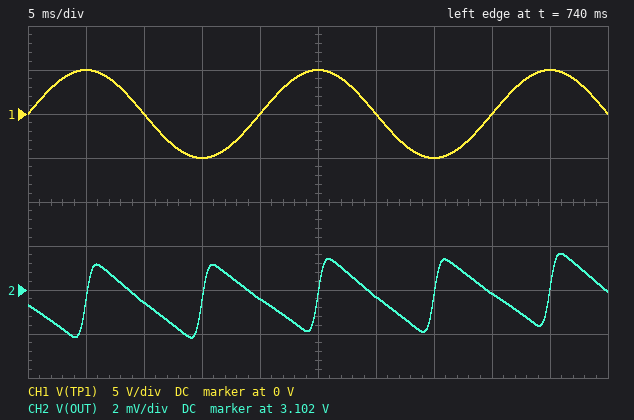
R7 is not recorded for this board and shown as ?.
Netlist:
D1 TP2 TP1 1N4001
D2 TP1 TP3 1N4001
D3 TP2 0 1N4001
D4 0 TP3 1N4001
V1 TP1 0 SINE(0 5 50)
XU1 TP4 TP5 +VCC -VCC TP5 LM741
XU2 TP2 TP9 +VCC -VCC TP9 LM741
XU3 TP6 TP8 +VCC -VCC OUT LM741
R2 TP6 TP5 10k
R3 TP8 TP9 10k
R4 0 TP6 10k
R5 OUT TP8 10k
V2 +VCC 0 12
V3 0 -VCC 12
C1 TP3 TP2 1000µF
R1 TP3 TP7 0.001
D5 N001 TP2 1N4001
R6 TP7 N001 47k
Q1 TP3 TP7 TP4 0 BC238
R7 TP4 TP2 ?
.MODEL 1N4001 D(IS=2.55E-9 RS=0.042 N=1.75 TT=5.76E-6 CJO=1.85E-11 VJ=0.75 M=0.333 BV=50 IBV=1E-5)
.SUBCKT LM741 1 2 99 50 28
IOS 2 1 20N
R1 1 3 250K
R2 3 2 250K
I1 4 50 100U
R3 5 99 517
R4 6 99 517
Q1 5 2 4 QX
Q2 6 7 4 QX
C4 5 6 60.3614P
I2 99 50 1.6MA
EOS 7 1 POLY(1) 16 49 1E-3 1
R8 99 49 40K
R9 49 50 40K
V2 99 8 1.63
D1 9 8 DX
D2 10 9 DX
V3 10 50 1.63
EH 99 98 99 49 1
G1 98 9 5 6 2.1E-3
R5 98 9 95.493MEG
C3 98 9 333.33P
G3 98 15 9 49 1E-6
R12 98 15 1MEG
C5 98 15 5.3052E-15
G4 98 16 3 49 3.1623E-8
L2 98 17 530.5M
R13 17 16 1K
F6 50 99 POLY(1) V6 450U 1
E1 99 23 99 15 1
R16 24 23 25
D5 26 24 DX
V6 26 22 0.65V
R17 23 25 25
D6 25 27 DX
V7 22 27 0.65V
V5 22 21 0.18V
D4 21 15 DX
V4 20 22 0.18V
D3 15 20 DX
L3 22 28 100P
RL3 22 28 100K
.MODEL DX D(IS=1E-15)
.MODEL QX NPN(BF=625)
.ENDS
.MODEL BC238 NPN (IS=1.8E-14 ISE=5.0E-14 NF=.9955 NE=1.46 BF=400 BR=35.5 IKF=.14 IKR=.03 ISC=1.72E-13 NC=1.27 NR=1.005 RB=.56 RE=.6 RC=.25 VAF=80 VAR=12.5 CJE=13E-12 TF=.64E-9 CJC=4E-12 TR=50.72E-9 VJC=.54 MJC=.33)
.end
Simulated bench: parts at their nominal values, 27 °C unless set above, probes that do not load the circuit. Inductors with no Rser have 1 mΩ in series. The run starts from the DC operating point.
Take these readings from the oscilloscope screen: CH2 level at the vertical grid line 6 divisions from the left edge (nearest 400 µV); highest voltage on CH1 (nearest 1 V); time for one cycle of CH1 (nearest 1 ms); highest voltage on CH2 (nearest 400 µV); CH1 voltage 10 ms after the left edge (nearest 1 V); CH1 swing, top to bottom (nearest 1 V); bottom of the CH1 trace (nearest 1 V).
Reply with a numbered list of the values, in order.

1. 3.1016 V
2. 5 V
3. 20 ms
4. 3.1036 V
5. 0 V
6. 10 V
7. -5 V
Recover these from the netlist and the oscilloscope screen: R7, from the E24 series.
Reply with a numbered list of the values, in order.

1. 9.1 kΩ
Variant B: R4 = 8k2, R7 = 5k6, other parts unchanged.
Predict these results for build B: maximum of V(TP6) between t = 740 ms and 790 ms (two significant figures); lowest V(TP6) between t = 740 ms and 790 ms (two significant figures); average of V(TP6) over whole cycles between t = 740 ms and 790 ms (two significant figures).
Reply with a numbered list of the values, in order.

1. 1.7 V
2. -580 mV
3. 300 mV
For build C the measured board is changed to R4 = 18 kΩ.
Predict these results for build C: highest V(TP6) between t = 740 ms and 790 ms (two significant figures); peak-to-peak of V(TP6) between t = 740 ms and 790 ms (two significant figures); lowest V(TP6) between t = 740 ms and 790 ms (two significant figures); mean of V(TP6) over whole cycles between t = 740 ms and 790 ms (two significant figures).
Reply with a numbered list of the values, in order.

1. 2.4 V
2. 3.2 V
3. -810 mV
4. 440 mV
